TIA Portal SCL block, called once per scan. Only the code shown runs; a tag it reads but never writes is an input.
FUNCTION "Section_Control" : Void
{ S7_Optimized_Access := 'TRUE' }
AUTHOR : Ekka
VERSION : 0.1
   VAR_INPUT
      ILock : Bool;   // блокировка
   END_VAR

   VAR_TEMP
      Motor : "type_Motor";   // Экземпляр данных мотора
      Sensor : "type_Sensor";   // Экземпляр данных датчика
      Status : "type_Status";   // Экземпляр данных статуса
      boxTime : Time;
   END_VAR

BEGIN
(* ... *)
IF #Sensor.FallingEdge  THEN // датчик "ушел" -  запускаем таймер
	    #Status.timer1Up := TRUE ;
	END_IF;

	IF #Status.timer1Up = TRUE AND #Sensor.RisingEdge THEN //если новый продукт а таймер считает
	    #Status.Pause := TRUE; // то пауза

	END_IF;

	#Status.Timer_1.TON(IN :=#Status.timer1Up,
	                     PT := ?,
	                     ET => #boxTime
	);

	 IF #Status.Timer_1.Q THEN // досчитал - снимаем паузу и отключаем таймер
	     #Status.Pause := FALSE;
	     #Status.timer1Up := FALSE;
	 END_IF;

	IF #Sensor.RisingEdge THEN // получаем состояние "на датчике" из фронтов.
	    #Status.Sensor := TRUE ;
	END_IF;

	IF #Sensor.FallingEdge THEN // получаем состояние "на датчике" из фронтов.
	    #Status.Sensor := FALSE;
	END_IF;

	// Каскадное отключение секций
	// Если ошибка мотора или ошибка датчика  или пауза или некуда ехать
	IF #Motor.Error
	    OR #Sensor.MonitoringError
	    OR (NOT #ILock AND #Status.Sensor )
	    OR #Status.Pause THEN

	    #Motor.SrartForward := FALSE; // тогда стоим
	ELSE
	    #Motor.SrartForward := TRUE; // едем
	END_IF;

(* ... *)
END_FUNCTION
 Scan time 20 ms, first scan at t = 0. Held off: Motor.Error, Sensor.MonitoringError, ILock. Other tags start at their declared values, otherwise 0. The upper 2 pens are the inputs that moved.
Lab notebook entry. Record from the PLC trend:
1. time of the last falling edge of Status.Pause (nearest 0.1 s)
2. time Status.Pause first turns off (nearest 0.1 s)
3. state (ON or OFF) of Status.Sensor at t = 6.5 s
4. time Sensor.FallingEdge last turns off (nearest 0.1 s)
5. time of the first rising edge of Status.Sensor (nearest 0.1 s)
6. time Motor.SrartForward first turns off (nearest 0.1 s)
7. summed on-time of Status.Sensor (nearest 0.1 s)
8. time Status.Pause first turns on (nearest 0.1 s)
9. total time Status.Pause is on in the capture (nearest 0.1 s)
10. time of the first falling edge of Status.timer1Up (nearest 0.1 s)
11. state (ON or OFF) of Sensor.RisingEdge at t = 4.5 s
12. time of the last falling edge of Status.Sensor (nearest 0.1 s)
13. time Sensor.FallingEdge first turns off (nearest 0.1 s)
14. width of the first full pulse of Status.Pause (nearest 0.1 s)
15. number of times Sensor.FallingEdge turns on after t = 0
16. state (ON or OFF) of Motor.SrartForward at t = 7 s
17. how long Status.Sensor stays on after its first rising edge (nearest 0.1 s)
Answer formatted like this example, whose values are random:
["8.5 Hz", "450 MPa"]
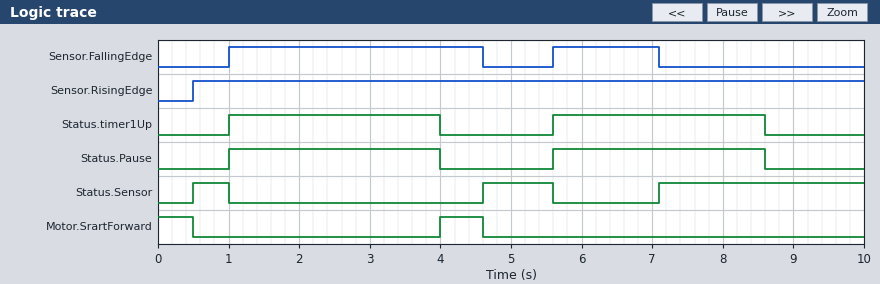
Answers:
["8.6 s", "4.0 s", "OFF", "7.1 s", "0.5 s", "0.5 s", "4.4 s", "1.0 s", "6.0 s", "4.0 s", "ON", "5.6 s", "4.6 s", "3.0 s", "2", "OFF", "0.5 s"]
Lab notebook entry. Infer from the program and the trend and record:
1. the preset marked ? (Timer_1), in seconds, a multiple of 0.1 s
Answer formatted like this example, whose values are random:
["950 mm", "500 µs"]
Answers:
["3.0 s"]
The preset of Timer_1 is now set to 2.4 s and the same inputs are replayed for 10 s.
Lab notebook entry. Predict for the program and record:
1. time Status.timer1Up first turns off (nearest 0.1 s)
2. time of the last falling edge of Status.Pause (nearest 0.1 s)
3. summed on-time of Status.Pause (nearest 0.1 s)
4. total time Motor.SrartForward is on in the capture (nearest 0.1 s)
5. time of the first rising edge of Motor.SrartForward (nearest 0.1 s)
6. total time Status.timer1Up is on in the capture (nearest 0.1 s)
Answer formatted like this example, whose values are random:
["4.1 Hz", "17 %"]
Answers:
["3.4 s", "8.0 s", "4.8 s", "1.7 s", "3.4 s", "4.8 s"]
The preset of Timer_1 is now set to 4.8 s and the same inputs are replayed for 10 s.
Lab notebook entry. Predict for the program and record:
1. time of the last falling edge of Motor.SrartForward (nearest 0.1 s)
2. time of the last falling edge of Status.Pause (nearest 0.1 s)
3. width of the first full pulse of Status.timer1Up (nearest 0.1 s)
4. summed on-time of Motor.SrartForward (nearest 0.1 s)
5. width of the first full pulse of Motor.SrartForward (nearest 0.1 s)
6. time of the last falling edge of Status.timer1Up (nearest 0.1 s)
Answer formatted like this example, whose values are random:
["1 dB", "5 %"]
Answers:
["7.1 s", "5.8 s", "4.8 s", "1.8 s", "1.3 s", "5.8 s"]
